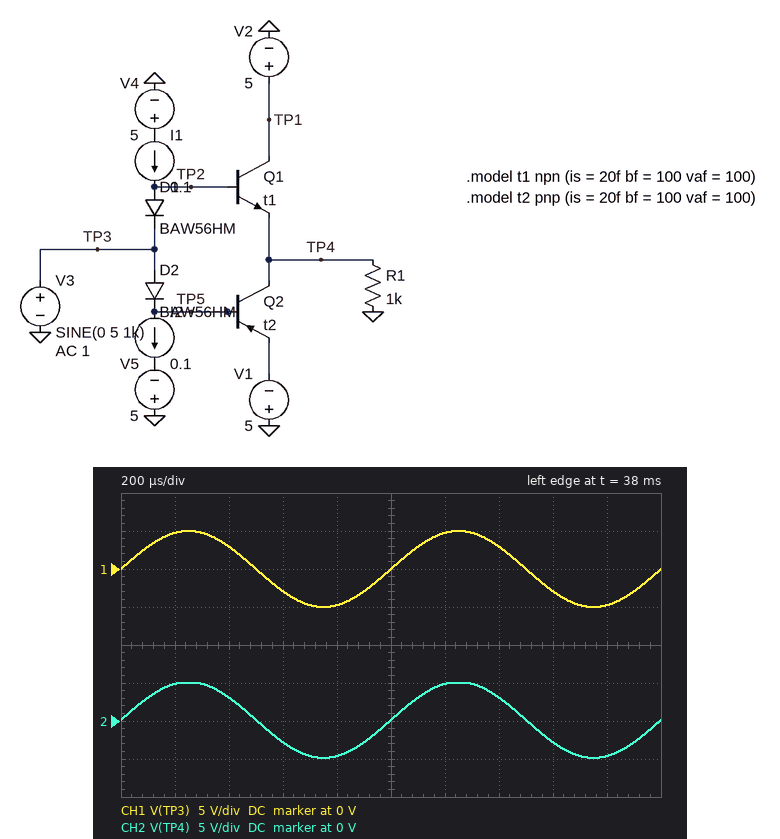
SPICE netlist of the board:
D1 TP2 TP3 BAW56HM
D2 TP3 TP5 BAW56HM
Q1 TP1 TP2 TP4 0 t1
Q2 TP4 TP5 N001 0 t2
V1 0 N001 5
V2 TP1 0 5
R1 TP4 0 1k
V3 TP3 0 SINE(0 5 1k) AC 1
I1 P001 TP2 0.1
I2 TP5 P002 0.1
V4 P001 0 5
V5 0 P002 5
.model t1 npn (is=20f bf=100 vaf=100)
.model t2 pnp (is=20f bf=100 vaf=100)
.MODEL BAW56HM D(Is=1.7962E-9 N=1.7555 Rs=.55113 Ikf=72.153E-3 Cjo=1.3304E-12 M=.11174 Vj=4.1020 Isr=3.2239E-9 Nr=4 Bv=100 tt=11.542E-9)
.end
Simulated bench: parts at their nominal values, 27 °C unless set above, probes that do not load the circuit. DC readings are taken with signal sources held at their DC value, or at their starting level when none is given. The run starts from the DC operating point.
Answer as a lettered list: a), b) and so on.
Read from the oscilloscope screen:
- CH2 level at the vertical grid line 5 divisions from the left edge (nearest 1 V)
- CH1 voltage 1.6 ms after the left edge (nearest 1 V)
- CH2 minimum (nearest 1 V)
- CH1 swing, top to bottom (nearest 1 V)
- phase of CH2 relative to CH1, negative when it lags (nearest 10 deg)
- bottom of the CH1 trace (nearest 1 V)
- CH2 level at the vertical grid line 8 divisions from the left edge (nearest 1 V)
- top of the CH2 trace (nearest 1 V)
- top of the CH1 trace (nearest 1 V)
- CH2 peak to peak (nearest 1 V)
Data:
a) 0 V
b) -3 V
c) -5 V
d) 10 V
e) 0 deg
f) -5 V
g) -3 V
h) 5 V
i) 5 V
j) 10 V
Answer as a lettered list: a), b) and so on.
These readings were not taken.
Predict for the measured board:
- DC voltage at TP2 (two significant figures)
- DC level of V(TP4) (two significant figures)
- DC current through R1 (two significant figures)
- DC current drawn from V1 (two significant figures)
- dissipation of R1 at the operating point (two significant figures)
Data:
a) 910 mV
b) 140 mV
c) 140 µA
d) 98 mA
e) 20 µW
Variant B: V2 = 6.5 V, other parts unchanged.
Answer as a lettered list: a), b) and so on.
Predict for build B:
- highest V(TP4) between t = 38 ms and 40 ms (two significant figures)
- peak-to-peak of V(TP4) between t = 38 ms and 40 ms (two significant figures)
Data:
a) 5.1 V
b) 10 V
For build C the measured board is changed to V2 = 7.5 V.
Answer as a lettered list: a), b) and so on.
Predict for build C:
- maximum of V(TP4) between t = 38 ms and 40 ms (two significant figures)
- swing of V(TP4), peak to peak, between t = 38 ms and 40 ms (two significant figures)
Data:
a) 5.1 V
b) 10 V
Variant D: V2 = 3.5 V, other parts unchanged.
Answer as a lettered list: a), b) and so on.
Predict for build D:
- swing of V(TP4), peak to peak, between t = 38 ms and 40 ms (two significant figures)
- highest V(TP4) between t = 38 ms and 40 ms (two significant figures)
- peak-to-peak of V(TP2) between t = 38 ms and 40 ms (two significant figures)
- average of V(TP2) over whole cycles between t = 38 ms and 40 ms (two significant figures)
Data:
a) 8.4 V
b) 3.5 V
c) 8.3 V
d) 620 mV
